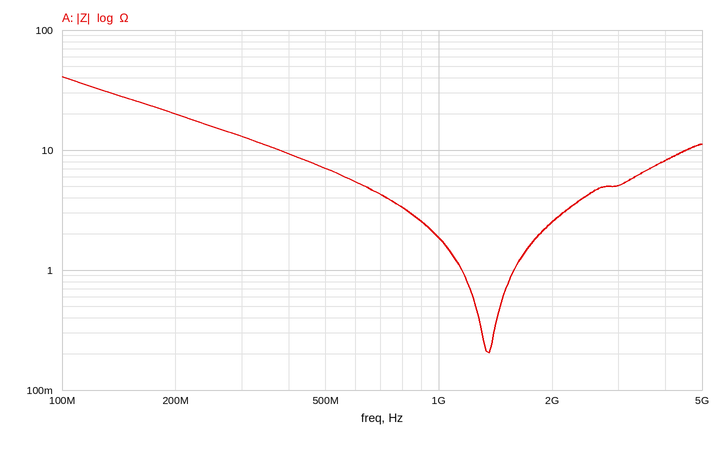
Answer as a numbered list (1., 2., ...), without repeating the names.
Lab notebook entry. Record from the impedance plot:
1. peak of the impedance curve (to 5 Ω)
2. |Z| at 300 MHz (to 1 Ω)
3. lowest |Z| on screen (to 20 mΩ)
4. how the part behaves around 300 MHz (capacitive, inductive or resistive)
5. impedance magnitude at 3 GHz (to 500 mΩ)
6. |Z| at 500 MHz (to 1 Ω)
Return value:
1. 40 Ω
2. 13 Ω
3. 200 mΩ
4. capacitive
5. 5.0 Ω
6. 7 Ω
